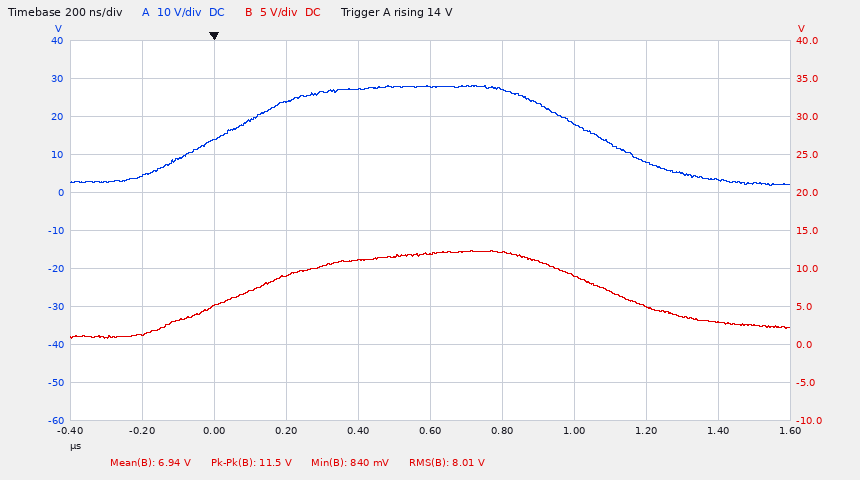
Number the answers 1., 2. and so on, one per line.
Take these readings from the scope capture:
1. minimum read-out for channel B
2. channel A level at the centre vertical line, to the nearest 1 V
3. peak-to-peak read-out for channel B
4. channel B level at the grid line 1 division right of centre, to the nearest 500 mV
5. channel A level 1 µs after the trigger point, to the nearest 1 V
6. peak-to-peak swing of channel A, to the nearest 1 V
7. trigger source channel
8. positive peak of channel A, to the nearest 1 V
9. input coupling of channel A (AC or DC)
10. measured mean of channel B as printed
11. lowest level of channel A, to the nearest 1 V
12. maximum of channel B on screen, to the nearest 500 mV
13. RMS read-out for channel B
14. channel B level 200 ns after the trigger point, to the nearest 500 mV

1. 840 mV
2. 28 V
3. 11.5 V
4. 12.0 V
5. 18 V
6. 26 V
7. channel A
8. 28 V
9. DC
10. 6.94 V
11. 2 V
12. 12.5 V
13. 8.01 V
14. 9.0 V
